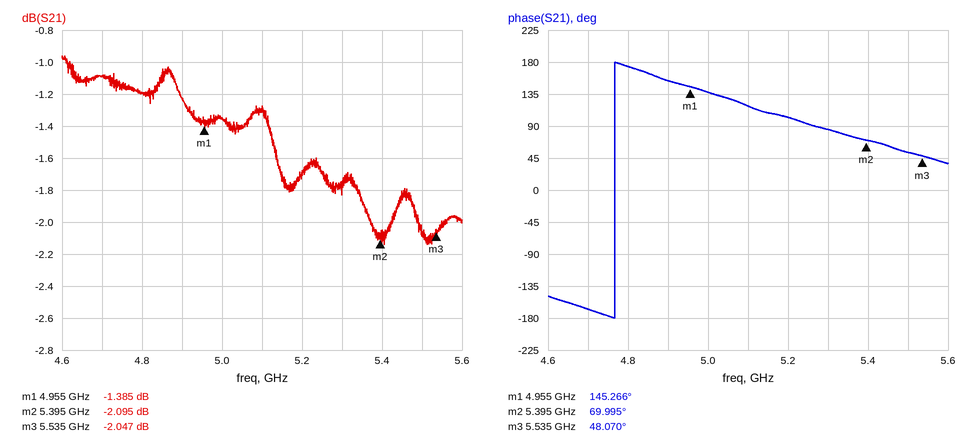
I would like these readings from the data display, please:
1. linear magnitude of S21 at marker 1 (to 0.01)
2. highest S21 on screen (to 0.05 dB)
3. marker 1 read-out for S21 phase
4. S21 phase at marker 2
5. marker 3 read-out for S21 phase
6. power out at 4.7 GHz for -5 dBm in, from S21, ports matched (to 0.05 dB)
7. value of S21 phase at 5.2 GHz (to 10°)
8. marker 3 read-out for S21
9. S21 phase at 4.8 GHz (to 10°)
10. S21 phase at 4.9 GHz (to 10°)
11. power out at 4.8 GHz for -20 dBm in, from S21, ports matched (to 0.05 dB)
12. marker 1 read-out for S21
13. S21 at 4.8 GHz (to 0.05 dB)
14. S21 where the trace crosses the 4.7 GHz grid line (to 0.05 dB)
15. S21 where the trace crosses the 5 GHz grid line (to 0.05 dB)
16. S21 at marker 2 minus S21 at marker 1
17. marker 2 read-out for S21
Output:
0.85
-0.95 dB
145.266°
69.995°
48.070°
-6.10 dBm
100°
-2.047 dB
170°
150°
-21.20 dBm
-1.385 dB
-1.20 dB
-1.10 dB
-1.35 dB
-0.710 dB
-2.095 dB
